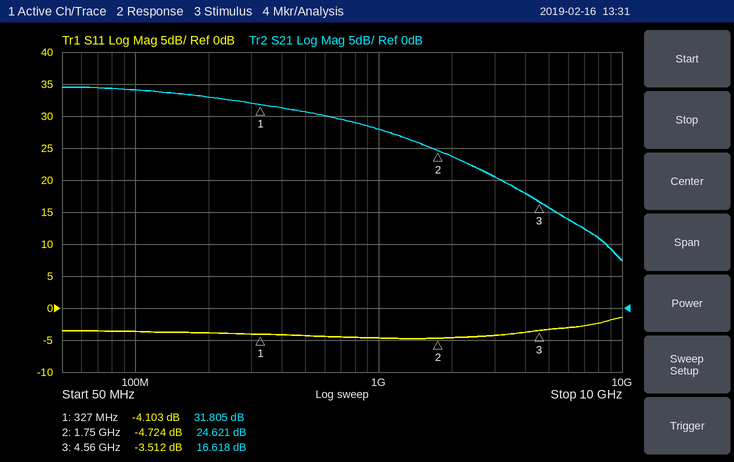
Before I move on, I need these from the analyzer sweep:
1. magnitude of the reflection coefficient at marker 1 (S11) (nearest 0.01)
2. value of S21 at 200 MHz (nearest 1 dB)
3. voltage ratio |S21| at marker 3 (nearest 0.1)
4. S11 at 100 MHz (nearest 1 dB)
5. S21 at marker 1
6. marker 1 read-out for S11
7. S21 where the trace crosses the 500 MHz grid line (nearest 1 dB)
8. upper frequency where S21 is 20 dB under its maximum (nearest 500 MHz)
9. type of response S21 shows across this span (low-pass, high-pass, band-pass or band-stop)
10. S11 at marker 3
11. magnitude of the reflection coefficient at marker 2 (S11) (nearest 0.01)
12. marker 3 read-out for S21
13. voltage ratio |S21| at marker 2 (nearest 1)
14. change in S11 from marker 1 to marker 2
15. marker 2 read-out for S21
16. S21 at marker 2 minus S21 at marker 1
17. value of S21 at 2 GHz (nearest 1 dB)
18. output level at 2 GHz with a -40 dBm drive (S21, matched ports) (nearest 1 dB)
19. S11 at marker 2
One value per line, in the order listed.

0.62
33 dB
6.8
-4 dB
31.805 dB
-4.103 dB
31 dB
5.5 GHz
low-pass
-3.512 dB
0.58
16.618 dB
17
-0.621 dB
24.621 dB
-7.184 dB
24 dB
-16 dBm
-4.724 dB
